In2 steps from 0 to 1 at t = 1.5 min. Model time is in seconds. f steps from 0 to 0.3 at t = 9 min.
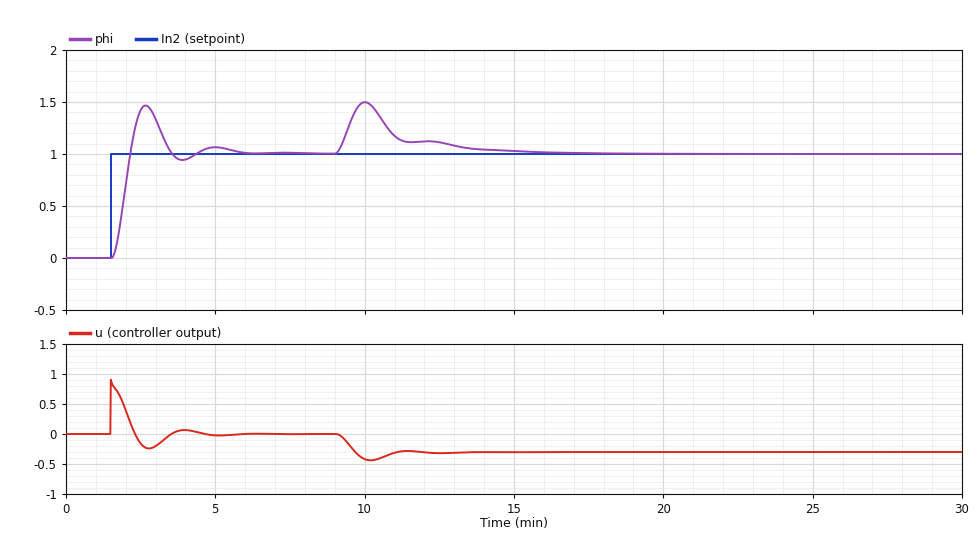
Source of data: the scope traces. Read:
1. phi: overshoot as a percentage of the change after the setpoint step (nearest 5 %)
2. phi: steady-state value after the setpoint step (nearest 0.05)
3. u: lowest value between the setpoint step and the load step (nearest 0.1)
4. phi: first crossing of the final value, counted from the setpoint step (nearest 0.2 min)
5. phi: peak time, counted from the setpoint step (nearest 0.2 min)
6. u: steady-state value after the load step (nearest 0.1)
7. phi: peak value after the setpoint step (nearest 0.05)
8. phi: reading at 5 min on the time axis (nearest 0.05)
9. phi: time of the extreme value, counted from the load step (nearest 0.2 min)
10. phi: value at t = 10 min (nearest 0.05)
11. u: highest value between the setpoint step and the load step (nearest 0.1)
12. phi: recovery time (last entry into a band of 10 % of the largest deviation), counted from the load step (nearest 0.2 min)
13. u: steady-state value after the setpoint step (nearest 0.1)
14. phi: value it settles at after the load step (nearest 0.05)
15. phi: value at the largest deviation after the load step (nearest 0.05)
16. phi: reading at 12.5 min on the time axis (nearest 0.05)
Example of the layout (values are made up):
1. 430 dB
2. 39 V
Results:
1. 45 %
2. 1.00
3. -0.2
4. 0.6 min
5. 1.2 min
6. -0.3
7. 1.45
8. 1.05
9. 1.0 min
10. 1.50
11. 0.9
12. 4.6 min
13. 0.0
14. 1.00
15. 1.50
16. 1.10
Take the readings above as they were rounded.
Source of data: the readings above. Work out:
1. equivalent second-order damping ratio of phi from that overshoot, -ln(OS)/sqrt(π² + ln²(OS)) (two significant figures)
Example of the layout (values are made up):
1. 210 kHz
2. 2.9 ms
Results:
1. 0.25
